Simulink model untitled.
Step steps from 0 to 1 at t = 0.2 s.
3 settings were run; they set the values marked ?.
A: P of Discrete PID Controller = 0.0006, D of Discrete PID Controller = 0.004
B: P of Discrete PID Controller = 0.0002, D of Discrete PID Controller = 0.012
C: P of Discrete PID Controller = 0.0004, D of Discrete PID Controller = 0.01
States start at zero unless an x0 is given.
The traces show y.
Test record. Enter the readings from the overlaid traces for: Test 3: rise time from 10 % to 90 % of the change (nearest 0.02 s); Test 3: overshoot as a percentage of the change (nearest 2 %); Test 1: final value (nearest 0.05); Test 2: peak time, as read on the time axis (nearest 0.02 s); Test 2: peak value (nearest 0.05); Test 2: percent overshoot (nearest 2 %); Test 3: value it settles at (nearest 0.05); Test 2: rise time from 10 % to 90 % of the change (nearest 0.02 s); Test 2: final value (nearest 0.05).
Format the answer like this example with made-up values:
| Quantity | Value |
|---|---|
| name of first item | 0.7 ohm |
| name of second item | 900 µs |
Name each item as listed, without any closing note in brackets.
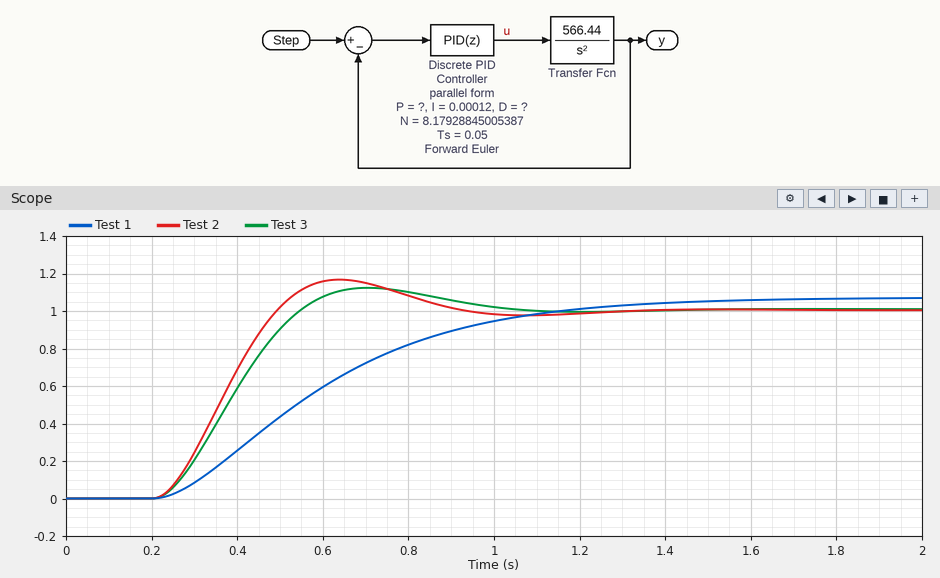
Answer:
| Quantity | Value |
|---|---|
| Test 3: rise time from 10 % to 90 % of the change | 0.24 s |
| Test 3: overshoot as a percentage of the change | 10 % |
| Test 1: final value | 1.05 |
| Test 2: peak time, as read on the time axis | 0.64 s |
| Test 2: peak value | 1.15 |
| Test 2: percent overshoot | 16 % |
| Test 3: value it settles at | 1.00 |
| Test 2: rise time from 10 % to 90 % of the change | 0.20 s |
| Test 2: final value | 1.00 |
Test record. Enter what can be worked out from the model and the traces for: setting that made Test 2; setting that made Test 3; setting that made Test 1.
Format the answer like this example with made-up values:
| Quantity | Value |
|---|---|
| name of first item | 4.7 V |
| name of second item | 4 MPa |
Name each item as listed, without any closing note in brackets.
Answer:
| Quantity | Value |
|---|---|
| setting that made Test 2 | B |
| setting that made Test 3 | C |
| setting that made Test 1 | A |
